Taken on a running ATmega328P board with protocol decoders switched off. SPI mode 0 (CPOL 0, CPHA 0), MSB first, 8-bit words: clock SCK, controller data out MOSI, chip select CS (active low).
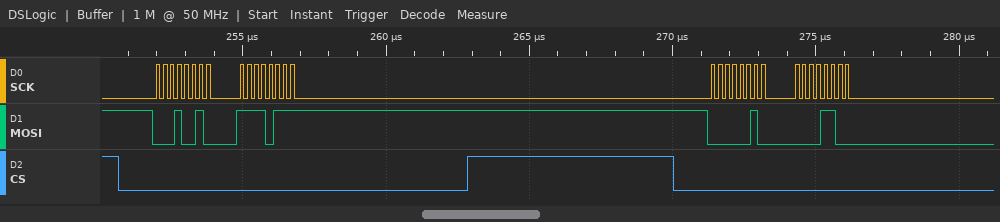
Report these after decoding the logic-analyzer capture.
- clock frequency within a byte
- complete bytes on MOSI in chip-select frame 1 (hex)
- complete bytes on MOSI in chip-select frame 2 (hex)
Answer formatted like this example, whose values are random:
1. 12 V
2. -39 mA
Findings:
1. 4 MHz
2. 12 F7
3. 02 0C
